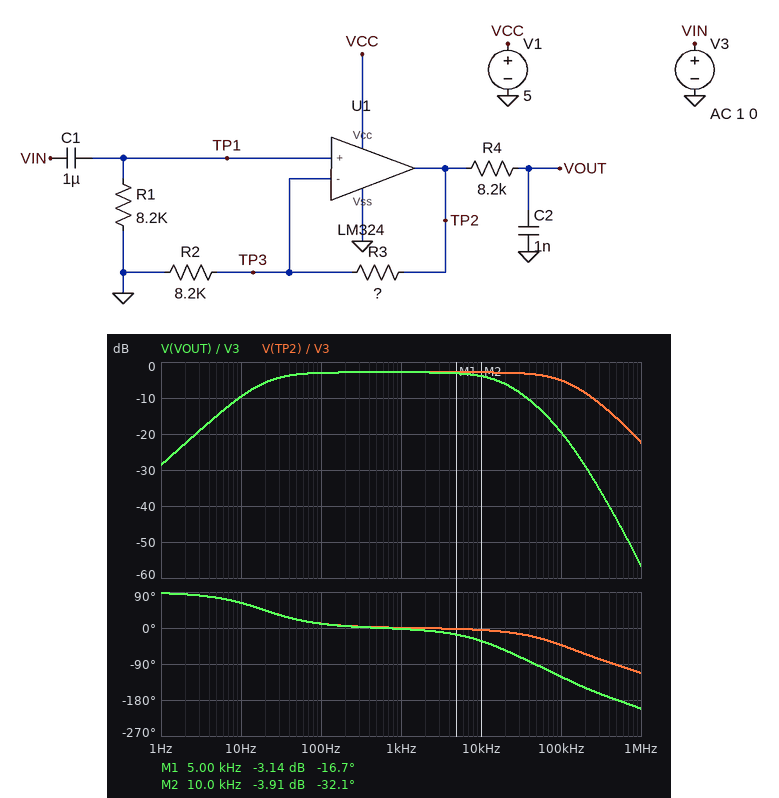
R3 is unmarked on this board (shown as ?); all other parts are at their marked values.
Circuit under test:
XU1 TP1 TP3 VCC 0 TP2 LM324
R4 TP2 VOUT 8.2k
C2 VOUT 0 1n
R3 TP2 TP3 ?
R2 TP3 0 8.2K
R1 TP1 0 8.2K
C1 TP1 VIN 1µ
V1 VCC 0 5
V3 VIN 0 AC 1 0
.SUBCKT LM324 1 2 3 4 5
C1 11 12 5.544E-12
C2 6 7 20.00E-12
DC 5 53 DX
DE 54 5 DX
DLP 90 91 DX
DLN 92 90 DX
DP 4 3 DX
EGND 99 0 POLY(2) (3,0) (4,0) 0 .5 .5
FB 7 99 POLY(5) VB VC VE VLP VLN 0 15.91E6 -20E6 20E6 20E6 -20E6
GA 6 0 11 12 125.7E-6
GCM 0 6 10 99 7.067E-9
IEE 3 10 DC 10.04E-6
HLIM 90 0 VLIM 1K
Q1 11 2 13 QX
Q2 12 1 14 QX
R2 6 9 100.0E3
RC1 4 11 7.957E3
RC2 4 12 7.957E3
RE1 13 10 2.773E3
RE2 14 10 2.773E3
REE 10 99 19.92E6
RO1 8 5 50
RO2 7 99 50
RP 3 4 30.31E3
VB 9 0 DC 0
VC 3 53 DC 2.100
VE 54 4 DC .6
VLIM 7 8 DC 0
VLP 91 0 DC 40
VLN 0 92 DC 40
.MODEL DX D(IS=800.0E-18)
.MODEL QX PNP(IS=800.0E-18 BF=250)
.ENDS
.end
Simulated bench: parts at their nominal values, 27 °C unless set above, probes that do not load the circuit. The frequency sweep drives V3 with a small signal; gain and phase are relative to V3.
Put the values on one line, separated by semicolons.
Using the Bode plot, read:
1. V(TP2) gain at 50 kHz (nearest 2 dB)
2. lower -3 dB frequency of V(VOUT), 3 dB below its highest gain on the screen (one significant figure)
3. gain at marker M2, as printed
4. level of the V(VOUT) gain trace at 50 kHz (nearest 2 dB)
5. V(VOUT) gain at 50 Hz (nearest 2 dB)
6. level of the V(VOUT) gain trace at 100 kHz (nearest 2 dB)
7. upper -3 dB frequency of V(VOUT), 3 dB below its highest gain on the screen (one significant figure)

-4 dB; 20 Hz; -3.91 dB; -12 dB; -4 dB; -20 dB; 20 kHz
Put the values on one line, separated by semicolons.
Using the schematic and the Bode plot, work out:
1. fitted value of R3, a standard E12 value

6.8 kΩ
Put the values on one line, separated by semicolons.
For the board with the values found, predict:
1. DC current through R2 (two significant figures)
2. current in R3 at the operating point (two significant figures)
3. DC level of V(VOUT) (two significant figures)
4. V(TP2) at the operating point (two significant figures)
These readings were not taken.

2.6 µA; 2.6 µA; 39 mV; 39 mV
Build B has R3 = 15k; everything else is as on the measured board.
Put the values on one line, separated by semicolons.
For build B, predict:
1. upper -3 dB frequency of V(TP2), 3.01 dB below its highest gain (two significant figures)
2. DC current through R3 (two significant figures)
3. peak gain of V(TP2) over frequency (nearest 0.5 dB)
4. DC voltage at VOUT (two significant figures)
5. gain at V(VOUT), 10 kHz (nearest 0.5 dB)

110 kHz; 2.0 µA; 0 dB; 46 mV; -1.0 dB
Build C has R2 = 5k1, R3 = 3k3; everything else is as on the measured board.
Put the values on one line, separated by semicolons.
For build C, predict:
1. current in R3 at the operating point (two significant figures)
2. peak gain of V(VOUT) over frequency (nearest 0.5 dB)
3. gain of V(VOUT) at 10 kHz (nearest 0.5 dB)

4.5 µA; -3.5 dB; -4.5 dB
